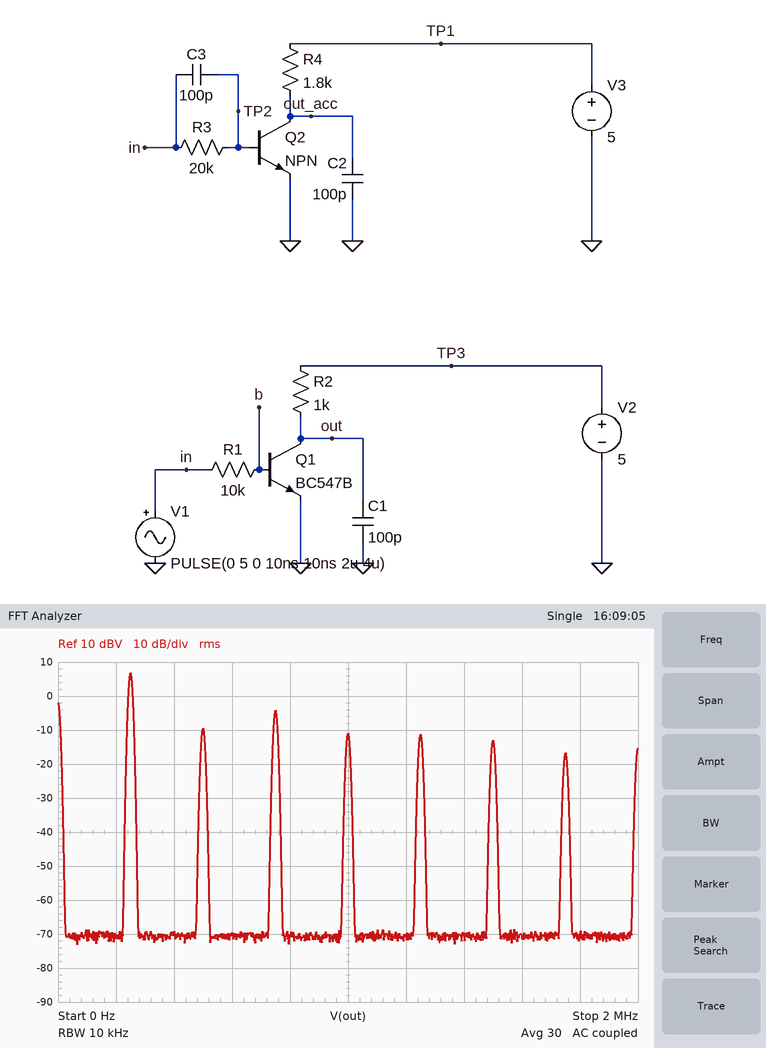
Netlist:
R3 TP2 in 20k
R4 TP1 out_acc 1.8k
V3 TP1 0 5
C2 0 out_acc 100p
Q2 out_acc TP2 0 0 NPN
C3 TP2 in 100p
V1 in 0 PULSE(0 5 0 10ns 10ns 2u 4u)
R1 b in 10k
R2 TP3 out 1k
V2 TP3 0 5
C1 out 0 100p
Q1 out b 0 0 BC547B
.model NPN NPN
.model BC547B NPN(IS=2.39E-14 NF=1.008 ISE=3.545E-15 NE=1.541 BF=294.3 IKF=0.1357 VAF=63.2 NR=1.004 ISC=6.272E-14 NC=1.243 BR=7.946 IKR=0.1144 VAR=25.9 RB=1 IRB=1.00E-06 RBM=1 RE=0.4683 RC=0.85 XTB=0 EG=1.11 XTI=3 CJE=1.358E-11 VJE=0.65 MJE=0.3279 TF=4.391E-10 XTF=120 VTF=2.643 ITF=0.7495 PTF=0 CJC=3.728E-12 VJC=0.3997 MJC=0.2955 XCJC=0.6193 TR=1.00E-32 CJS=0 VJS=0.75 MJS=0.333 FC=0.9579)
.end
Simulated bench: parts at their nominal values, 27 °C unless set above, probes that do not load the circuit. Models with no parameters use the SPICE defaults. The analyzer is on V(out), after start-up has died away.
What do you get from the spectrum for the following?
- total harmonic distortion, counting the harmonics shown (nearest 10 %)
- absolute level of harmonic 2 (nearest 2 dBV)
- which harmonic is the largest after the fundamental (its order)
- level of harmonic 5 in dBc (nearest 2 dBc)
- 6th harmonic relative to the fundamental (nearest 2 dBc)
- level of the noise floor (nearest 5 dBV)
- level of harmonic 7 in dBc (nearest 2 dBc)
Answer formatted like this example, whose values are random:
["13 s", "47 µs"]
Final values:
["40 %", "-10 dBV", "3", "-18 dBc", "-20 dBc", "-70 dBV", "-24 dBc"]
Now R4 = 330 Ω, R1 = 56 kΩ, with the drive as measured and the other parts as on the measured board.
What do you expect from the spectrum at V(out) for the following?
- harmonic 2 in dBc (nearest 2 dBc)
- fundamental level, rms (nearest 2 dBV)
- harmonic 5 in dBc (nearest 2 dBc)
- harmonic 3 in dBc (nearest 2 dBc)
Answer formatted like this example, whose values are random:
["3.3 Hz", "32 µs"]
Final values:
["-12 dBc", "6 dBV", "-20 dBc", "-14 dBc"]
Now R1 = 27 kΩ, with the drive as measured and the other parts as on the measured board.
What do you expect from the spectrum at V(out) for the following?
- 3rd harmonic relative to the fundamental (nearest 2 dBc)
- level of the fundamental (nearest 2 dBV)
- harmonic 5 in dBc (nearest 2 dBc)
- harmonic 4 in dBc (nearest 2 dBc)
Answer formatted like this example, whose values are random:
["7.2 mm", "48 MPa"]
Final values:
["-14 dBc", "6 dBV", "-20 dBc", "-16 dBc"]
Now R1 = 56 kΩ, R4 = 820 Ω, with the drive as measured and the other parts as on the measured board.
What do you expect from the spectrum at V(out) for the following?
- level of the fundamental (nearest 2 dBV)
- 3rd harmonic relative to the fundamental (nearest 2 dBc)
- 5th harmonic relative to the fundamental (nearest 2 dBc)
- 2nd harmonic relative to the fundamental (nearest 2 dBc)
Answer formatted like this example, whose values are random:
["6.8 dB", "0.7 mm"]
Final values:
["6 dBV", "-14 dBc", "-20 dBc", "-12 dBc"]
